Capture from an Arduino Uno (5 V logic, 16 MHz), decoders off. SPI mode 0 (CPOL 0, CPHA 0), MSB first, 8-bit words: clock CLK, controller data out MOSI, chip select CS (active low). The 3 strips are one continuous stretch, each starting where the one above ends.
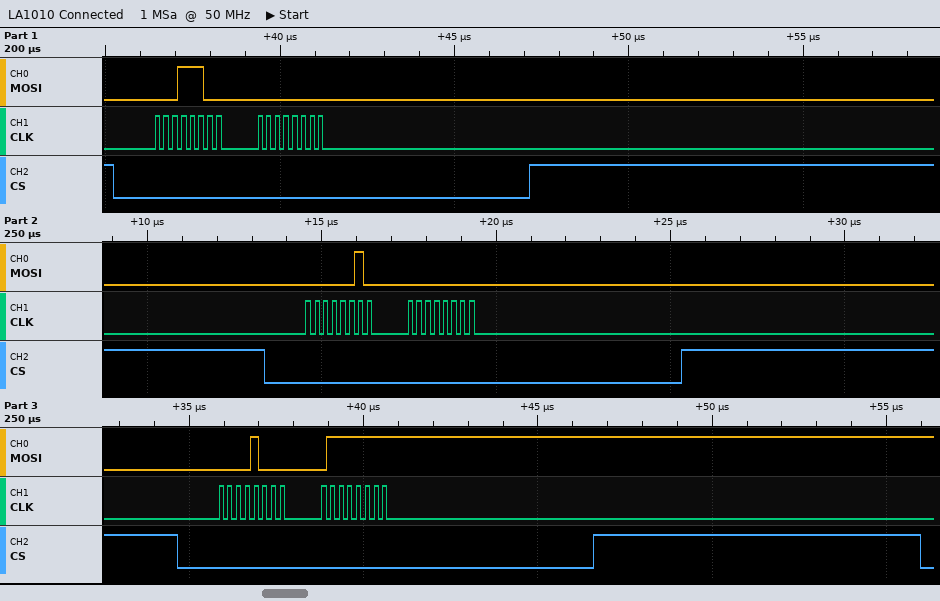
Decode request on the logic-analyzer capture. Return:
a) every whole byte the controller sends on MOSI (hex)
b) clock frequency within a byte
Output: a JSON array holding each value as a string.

["0x1C 0x00 0x02 0x00 0x08 0x7F", "4 MHz"]
